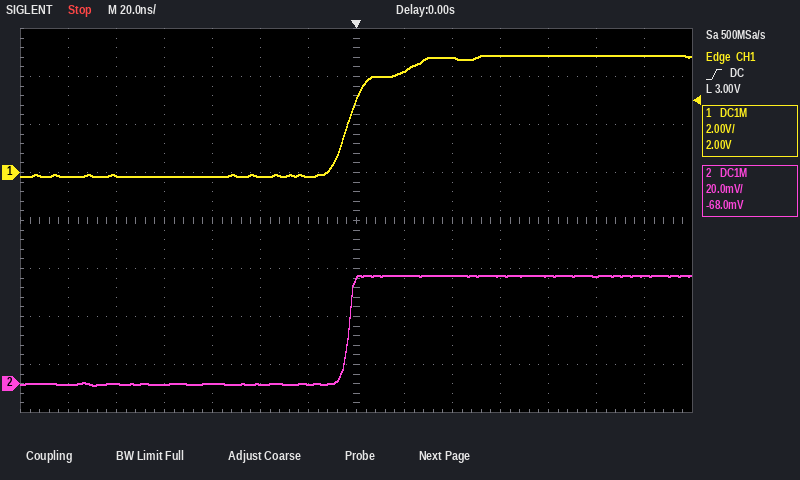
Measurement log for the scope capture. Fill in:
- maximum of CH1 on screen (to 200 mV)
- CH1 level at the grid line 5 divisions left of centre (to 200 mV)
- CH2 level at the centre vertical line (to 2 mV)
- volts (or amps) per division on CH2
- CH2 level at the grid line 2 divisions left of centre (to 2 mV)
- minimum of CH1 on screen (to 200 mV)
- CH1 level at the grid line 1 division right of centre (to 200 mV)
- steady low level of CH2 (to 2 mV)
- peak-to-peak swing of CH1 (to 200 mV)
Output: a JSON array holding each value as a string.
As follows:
["4.8 V", "-200 mV", "44 mV", "20 mV", "0 mV", "-200 mV", "4.2 V", "0 mV", "5.0 V"]
